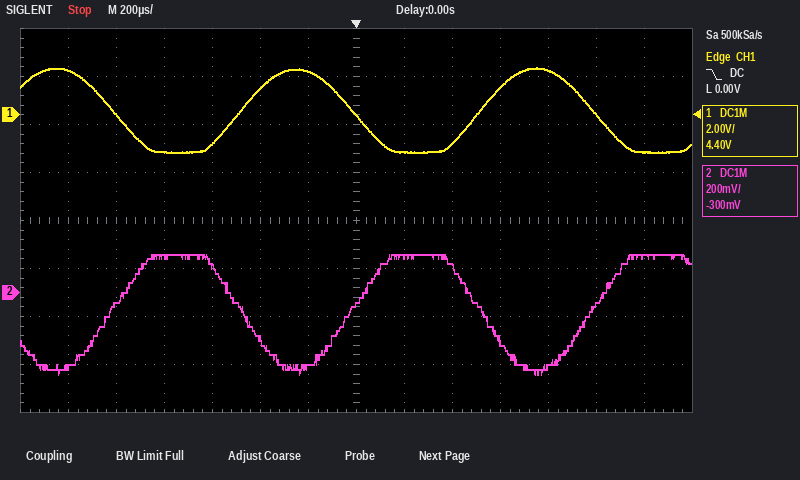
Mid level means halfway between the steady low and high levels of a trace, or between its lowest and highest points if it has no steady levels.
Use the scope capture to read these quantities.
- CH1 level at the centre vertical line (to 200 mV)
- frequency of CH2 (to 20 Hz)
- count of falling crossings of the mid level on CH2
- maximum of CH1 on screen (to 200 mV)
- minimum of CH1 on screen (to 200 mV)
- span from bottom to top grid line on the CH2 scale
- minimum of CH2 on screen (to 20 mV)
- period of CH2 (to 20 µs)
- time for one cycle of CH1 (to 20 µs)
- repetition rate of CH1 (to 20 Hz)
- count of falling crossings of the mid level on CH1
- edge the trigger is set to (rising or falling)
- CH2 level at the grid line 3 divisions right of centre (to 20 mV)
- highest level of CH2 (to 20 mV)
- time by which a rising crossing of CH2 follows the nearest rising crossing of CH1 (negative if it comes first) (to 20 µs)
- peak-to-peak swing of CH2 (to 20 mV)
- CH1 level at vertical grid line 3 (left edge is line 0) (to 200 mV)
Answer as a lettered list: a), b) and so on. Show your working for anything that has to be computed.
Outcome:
a) 0.0 V
b) 1 / 1.00 ms ≈ 1.00 kHz
c) 2
d) 2.0 V
e) -1.6 V
f) 1.6 V
g) -340 mV
h) 1.00 ms
i) 1.00 ms
j) 1 / 1.00 ms ≈ 1.00 kHz
k) 3
l) falling
m) -200 mV
n) 160 mV
o) +460 µs
p) 160 mV − (-340 mV) = 500 mV
q) -1.6 V
